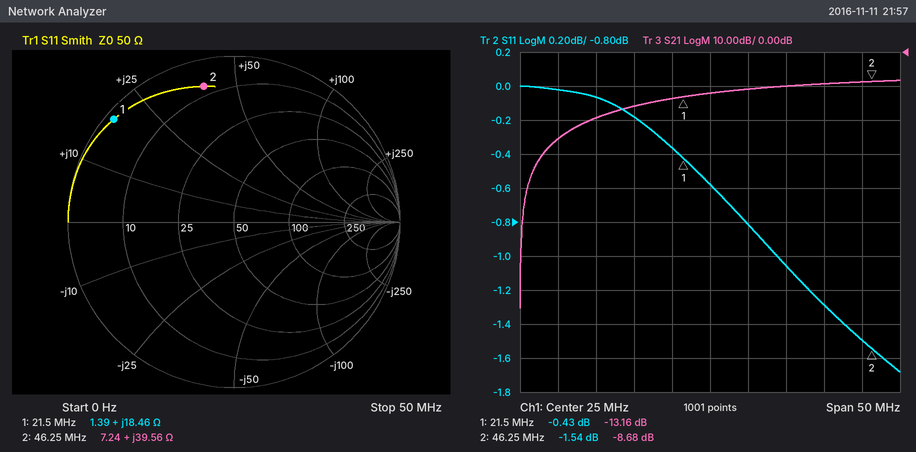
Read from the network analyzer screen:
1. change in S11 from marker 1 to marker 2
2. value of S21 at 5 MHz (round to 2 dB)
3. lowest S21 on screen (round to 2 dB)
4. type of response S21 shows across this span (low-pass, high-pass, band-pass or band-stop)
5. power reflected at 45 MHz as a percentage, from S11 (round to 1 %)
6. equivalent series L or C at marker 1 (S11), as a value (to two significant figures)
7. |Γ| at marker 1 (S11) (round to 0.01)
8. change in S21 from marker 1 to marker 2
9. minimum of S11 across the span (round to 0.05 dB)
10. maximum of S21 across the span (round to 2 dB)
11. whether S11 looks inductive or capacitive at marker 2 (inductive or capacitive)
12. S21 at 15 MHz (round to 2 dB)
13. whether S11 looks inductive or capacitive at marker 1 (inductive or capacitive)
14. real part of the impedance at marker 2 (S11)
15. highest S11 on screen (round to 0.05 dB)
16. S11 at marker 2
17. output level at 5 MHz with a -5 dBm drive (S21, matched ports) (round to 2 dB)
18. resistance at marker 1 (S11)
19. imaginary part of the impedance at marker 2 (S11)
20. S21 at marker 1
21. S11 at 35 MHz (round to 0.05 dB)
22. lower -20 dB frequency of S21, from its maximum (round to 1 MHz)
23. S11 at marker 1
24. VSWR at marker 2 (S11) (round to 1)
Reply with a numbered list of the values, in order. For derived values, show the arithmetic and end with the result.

1. -1.54 − (-0.43) = -1.11 dB
2. -26 dB
3. -76 dB
4. high-pass
5. 10^(-1.5/10) ≈ 71 %
6. L = 18.46 Ω/(2π × 21.5 MHz) ≈ 137 nH, so 140 nH to two significant figures
7. 0.95
8. -8.68 − (-13.16) = 4.48 dB
9. -1.70 dB
10. -8 dB
11. inductive
12. -16 dB
13. inductive
14. 7.24 Ω
15. 0.00 dB
16. -1.54 dB
17. -5 dBm + (-26 dB) = -30 dBm
18. 1.39 Ω
19. +39.56 Ω
20. -13.16 dB
21. -1.05 dB
22. 4 MHz
23. -0.43 dB
24. (1 + 0.8375)/(1 − 0.8375) ≈ 11
